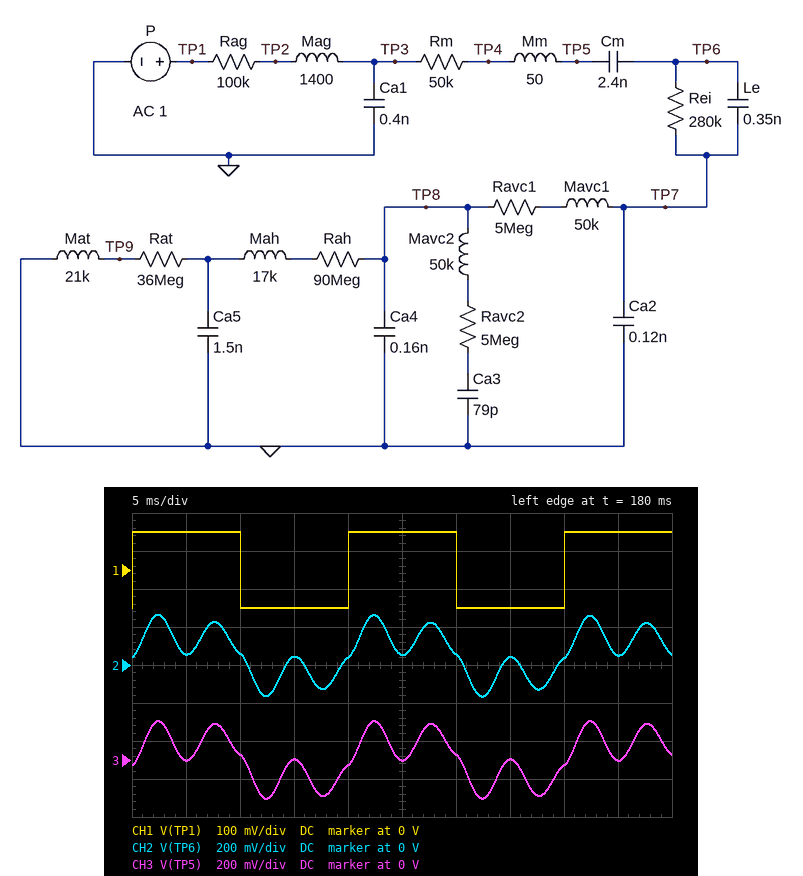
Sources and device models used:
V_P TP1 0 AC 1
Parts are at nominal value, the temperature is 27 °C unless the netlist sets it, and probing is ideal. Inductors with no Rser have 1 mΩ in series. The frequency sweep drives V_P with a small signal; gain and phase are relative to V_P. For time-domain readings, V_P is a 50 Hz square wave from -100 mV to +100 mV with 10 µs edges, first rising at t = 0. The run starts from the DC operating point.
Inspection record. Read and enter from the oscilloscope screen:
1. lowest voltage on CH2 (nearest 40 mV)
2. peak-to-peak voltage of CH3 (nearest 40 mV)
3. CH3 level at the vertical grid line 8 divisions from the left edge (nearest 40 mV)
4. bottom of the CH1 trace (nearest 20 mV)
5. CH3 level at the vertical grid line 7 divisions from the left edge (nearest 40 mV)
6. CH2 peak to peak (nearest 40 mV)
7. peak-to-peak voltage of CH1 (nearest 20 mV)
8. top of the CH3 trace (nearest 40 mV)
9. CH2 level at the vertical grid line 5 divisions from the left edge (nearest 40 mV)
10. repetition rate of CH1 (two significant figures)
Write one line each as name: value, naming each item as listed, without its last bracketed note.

lowest voltage on CH2: -160 mV
peak-to-peak voltage of CH3: 400 mV
CH3 level at the vertical grid line 8 divisions from the left edge: -40 mV
bottom of the CH1 trace: -100 mV
CH3 level at the vertical grid line 7 divisions from the left edge: 0 V
CH2 peak to peak: 440 mV
peak-to-peak voltage of CH1: 200 mV
top of the CH3 trace: 200 mV
CH2 level at the vertical grid line 5 divisions from the left edge: 40 mV
repetition rate of CH1: 50 Hz
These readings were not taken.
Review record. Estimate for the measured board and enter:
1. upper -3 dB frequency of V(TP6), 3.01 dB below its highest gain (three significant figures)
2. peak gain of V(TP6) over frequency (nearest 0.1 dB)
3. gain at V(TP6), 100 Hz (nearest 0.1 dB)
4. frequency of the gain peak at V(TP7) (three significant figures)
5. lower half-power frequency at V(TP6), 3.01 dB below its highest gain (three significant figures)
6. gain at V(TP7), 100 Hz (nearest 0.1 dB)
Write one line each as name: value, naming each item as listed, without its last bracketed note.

upper -3 dB frequency of V(TP6), 3.01 dB below its highest gain: 196 Hz
peak gain of V(TP6) over frequency: 22.7 dB
gain at V(TP6), 100 Hz: 2.3 dB
frequency of the gain peak at V(TP7): 190 Hz
lower half-power frequency at V(TP6), 3.01 dB below its highest gain: 183 Hz
gain at V(TP7), 100 Hz: 2.3 dB
